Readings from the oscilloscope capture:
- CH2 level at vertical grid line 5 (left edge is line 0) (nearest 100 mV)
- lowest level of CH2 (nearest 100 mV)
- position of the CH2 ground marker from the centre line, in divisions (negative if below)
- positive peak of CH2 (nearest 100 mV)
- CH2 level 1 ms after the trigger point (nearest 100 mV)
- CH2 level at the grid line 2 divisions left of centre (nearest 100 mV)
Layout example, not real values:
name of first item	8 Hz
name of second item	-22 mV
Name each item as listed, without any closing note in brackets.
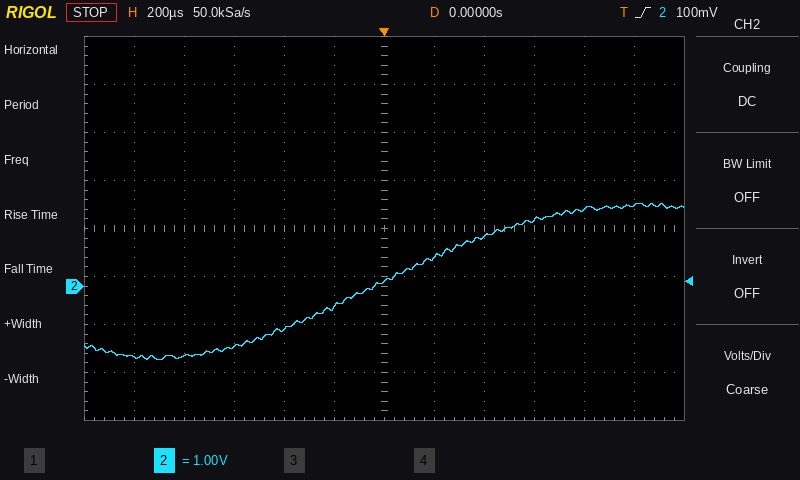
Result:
CH2 level at vertical grid line 5 (left edge is line 0)	-400 mV
lowest level of CH2	-1.5 V
position of the CH2 ground marker from the centre line, in divisions	-1.2 div
positive peak of CH2	1.7 V
CH2 level 1 ms after the trigger point	1.7 V
CH2 level at the grid line 2 divisions left of centre	-900 mV
